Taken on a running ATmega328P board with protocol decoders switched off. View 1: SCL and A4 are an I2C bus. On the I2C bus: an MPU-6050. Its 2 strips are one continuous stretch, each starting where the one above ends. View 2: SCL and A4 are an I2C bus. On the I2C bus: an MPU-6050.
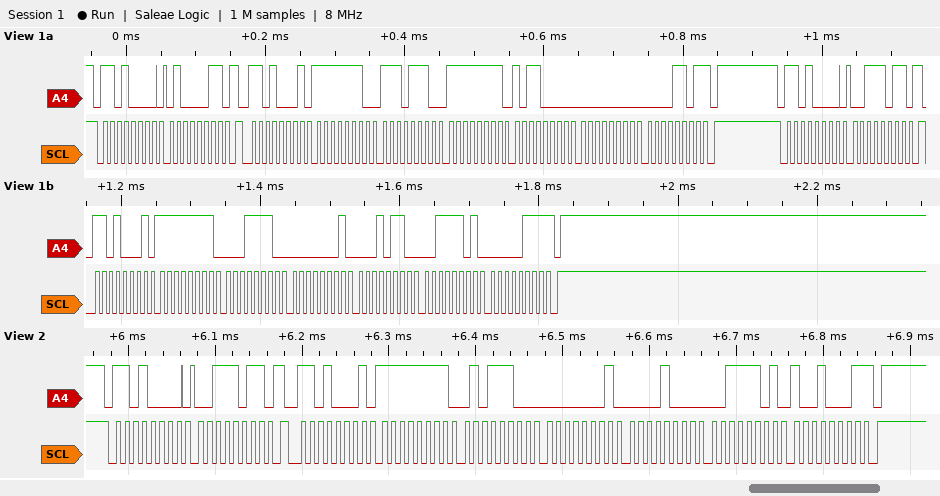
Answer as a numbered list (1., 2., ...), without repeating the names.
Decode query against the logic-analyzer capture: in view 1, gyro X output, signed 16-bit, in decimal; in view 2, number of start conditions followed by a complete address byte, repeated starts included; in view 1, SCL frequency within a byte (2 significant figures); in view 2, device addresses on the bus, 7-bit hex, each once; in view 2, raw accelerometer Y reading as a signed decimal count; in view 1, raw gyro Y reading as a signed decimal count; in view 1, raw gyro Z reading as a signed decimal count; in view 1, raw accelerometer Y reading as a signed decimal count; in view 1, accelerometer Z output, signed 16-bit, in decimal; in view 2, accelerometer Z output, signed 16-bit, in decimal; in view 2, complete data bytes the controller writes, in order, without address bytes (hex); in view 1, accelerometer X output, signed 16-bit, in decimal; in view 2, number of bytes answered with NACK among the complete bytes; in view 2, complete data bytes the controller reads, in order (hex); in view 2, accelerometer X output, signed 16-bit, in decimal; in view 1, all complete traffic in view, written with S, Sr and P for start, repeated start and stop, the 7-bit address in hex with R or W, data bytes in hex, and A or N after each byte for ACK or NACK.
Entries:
1. -274
2. 2
3. 100 kHz
4. 0x68
5. 264
6. -80
7. 13
8. 278
9. 15623
10. 15761
11. 3B
12. -226
13. 1
14. FF 5C 01 08 3D 91
15. -164
16. S 68W A 43 A Sr 68R A FE A EE A FF A B0 A 00 A 0D N P S 68W A 3B A Sr 68R A FF A 1E A 01 A 16 A 3D A 07 N P
